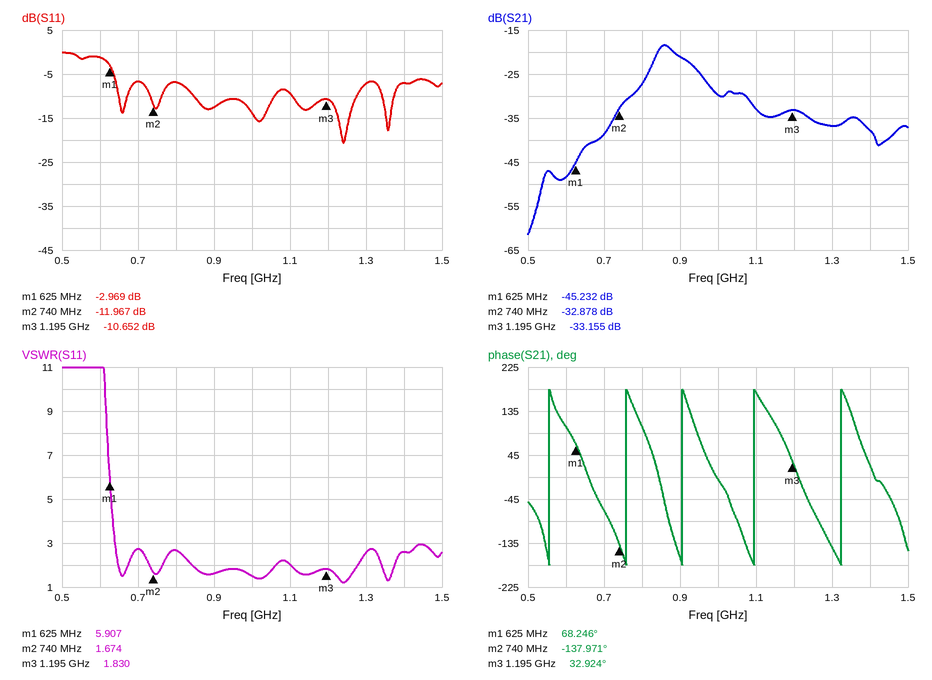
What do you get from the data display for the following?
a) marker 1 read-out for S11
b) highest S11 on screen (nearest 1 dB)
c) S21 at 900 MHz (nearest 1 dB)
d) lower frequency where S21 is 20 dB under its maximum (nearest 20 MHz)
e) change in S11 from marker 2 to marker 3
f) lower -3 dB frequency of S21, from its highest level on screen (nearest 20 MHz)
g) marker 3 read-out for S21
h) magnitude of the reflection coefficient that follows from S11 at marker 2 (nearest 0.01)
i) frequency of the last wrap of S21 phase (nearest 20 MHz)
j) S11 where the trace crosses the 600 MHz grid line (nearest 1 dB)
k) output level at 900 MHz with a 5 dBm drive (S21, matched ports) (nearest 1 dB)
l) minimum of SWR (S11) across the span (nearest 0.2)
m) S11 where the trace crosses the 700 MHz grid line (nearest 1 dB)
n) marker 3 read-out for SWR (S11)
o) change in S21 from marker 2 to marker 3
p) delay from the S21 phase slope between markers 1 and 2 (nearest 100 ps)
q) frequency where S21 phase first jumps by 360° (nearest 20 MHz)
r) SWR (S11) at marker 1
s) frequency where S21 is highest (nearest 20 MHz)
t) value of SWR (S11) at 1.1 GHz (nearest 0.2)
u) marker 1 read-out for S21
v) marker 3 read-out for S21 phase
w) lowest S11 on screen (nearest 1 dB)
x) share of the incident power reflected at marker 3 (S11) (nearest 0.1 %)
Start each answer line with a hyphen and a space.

- -2.969 dB
- 0 dB
- -21 dB
- 700 MHz
- 1.315 dB
- 840 MHz
- -33.155 dB
- 0.25
- 1.32 GHz
- -1 dB
- -16 dBm
- 1.2
- -7 dB
- 1.830
- -0.277 dB
- 5.0 ns
- 560 MHz
- 5.907
- 860 MHz
- 2.0
- -45.232 dB
- 32.924°
- -21 dB
- 8.6 %
